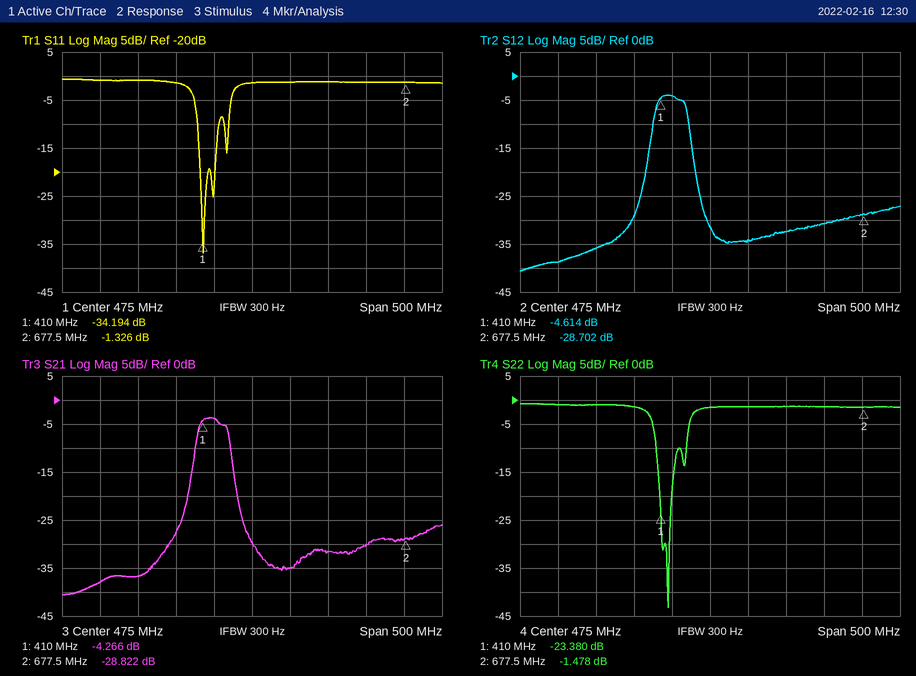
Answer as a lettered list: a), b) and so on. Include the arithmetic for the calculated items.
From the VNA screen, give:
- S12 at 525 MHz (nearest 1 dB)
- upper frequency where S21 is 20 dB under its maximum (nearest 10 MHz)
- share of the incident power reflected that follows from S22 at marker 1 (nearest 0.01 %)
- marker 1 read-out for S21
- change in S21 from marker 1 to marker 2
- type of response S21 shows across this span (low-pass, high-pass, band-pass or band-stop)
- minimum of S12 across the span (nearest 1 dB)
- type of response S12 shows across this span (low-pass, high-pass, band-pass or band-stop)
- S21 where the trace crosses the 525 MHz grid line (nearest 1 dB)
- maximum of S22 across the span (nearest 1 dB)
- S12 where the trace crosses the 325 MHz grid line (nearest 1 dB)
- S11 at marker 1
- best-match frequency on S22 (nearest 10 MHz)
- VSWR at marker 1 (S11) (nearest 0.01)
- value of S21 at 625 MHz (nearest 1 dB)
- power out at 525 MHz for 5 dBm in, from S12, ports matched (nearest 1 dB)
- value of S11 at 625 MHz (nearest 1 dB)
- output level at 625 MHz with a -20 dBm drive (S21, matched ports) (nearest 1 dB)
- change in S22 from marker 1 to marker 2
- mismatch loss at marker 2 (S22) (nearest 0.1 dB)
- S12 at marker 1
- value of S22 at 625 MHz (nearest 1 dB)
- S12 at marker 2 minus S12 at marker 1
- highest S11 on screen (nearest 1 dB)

a) -34 dB
b) 460 MHz
c) 10^(-23.38/10) ≈ 0.46 %
d) -4.266 dB
e) -28.822 − (-4.266) = -24.556 dB
f) band-pass
g) -41 dB
h) band-pass
i) -35 dB
j) -1 dB
k) -36 dB
l) -34.194 dB
m) 420 MHz
n) (1 + 0.0195)/(1 − 0.0195) ≈ 1.04
o) -30 dB
p) 5 dBm + (-34 dB) = -29 dBm
q) -1 dB
r) -20 dBm + (-30 dB) = -50 dBm
s) -1.478 − (-23.38) = 21.902 dB
t) −10 log10(1 − 10^(-1.478/10)) ≈ 5.4 dB
u) -4.614 dB
v) -1 dB
w) -28.702 − (-4.614) = -24.088 dB
x) -1 dB
